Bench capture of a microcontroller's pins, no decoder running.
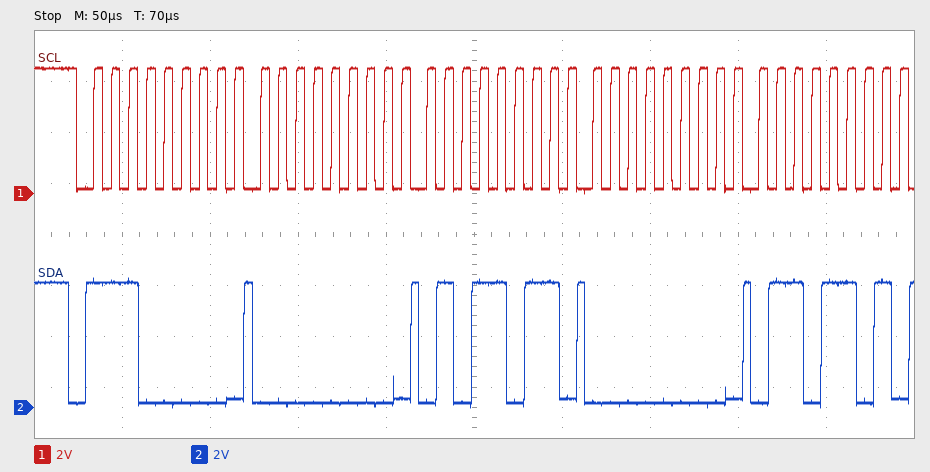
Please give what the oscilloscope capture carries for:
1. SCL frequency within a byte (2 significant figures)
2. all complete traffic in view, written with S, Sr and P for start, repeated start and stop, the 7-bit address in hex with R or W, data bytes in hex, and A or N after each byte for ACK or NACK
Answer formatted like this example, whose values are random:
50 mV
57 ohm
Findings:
100 kHz
S 70W A 00 A 5B A 00 A 6D A
